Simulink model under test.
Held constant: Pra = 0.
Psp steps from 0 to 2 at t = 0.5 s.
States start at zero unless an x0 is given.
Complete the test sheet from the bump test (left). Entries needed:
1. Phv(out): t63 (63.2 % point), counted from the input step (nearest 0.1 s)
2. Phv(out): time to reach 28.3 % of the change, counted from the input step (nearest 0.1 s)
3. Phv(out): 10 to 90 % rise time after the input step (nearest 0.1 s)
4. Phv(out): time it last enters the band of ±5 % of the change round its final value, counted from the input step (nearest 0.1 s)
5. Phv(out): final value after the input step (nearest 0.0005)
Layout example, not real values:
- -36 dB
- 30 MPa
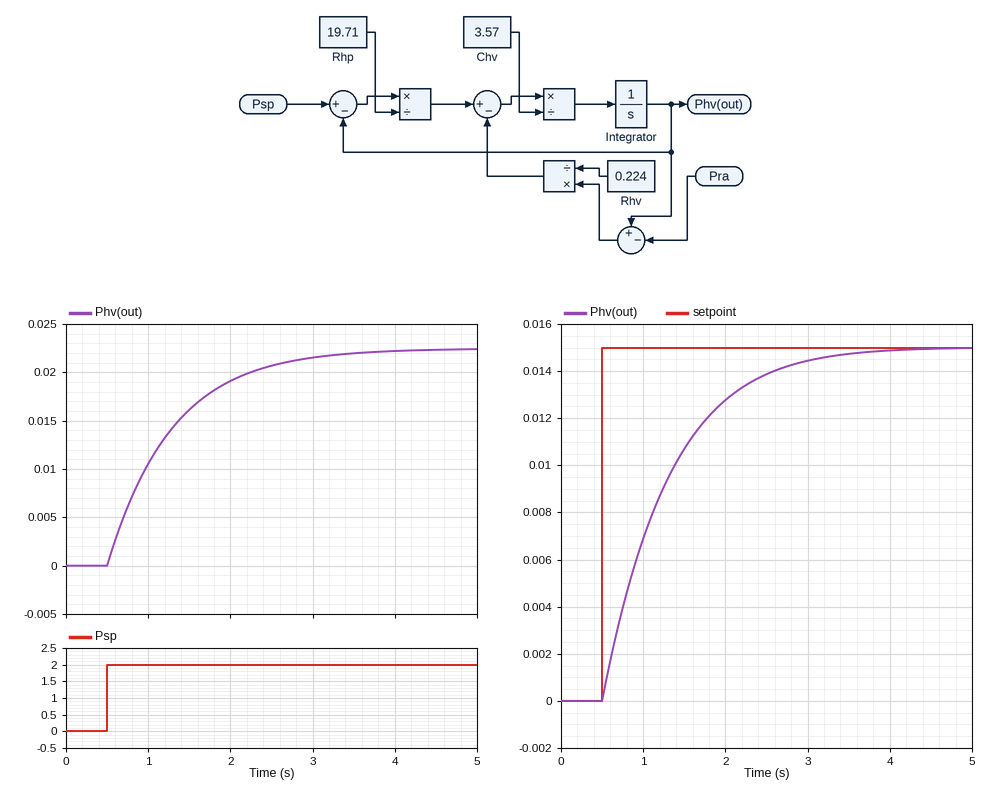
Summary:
- 0.8 s
- 0.3 s
- 1.7 s
- 2.4 s
- 0.0225
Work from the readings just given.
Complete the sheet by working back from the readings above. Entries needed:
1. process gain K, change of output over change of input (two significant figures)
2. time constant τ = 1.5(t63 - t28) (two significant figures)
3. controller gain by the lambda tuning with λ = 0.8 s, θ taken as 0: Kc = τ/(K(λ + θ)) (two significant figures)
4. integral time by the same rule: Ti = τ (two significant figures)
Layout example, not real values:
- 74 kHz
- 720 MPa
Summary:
- 0.011
- 0.75 s
- 85
- 0.75 s
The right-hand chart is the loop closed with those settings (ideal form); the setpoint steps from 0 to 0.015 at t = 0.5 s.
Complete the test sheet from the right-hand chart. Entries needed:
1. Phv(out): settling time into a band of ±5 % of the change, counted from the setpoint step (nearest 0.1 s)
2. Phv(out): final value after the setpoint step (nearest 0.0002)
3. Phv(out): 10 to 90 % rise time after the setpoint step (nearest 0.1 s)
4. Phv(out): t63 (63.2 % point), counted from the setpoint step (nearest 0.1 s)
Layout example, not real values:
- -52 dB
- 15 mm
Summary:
- 2.3 s
- 0.0150
- 1.7 s
- 0.8 s
